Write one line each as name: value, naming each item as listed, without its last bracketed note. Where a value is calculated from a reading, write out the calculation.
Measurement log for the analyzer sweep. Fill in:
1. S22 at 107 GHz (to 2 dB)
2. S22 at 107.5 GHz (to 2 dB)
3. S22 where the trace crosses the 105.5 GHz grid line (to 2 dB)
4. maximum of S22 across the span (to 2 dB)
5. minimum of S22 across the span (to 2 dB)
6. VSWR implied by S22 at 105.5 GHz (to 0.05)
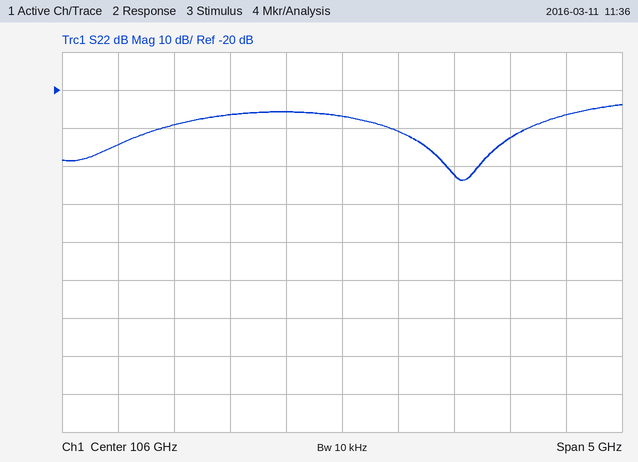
S22 at 107 GHz: -42 dB
S22 at 107.5 GHz: -32 dB
S22 where the trace crosses the 105.5 GHz grid line: -26 dB
maximum of S22 across the span: -24 dB
minimum of S22 across the span: -44 dB
VSWR implied by S22 at 105.5 GHz: |Γ| = 10^(-26/20) = 0.0501; VSWR = (1 + 0.0501)/(1 − 0.0501) ≈ 1.11, so 1.10 to the nearest 0.05
